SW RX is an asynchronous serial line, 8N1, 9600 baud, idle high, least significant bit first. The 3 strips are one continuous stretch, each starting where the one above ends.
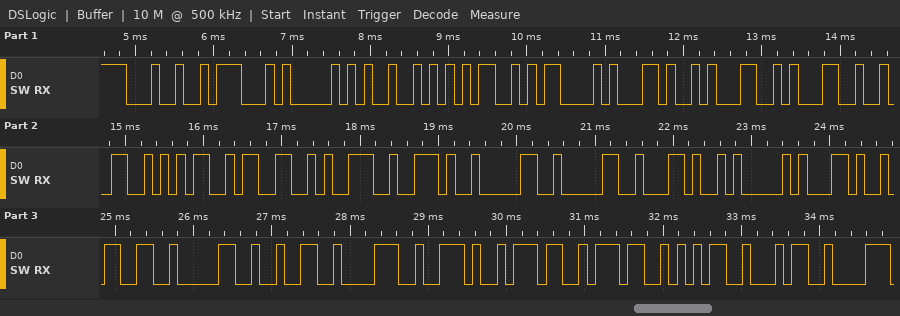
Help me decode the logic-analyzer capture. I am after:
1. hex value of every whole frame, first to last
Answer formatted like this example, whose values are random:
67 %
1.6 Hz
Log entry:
0x24 0x47 0x50 0x52 0x4D 0x43 0x2C 0x31 0x31 0x32 0x35 0x33 0x39 0x2E 0x30 0x30 0x2C 0x41 0x2C 0x33 0x30 0x32 0x38 0x2E 0x37 0x37 0x35 0x34
